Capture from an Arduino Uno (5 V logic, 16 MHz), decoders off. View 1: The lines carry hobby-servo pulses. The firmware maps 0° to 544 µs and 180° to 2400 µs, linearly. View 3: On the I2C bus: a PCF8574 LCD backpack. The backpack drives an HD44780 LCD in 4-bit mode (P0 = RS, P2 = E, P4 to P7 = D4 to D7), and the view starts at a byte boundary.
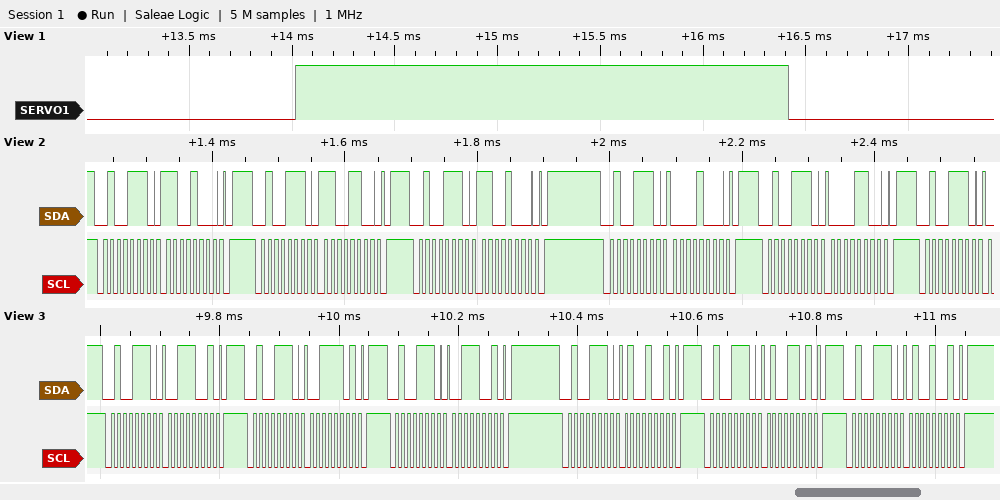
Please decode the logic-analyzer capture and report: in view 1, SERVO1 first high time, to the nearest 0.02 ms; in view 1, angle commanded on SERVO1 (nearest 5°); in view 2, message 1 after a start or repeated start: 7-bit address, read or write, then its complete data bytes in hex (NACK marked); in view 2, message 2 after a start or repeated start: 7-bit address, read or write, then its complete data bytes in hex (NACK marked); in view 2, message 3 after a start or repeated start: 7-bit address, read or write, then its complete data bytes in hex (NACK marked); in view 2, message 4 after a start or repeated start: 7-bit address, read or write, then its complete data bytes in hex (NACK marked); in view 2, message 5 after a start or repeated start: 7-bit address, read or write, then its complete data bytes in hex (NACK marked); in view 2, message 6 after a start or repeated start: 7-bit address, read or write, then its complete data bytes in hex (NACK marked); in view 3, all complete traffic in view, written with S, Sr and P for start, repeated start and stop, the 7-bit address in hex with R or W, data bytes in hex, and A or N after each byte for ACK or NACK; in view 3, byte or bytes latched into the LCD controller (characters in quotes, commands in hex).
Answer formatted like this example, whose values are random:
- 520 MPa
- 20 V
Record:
- 2.40 ms
- 180°
- 0x27 write: C8
- 0x27 write: CC
- 0x27 write: C8
- 0x27 write: 08
- 0x27 write: 0C
- 0x27 write
- S 27W A 39 A P S 27W A 3D A P S 27W A 39 A P S 27W A 49 A P S 27W A 4D A P S 27W A 49 A P
- '4'
